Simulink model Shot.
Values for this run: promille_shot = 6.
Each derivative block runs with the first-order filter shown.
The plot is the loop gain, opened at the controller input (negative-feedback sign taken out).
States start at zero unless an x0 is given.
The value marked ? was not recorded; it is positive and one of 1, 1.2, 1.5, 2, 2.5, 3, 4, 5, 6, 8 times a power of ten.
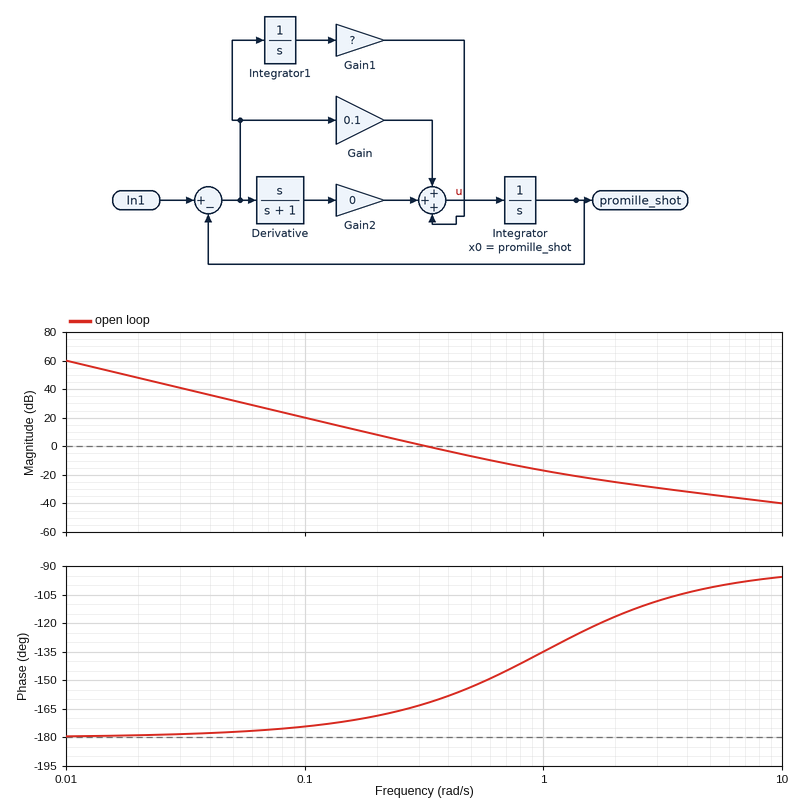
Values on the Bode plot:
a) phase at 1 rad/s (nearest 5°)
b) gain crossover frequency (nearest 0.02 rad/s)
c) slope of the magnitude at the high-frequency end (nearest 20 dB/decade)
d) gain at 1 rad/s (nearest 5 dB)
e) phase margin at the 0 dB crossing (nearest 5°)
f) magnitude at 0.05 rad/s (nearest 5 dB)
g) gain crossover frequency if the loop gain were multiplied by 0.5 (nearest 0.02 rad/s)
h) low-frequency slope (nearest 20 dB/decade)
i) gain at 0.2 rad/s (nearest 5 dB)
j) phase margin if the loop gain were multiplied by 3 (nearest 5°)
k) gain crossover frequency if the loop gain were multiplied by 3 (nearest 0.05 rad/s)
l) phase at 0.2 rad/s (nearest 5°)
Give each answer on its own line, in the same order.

-135°
0.32 rad/s
-20 dB/decade
-15 dB
20°
30 dB
0.22 rad/s
-40 dB/decade
10 dB
30°
0.60 rad/s
-170°
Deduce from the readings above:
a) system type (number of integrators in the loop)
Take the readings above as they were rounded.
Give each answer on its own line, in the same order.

2
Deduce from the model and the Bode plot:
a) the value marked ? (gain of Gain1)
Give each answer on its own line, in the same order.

0.1
